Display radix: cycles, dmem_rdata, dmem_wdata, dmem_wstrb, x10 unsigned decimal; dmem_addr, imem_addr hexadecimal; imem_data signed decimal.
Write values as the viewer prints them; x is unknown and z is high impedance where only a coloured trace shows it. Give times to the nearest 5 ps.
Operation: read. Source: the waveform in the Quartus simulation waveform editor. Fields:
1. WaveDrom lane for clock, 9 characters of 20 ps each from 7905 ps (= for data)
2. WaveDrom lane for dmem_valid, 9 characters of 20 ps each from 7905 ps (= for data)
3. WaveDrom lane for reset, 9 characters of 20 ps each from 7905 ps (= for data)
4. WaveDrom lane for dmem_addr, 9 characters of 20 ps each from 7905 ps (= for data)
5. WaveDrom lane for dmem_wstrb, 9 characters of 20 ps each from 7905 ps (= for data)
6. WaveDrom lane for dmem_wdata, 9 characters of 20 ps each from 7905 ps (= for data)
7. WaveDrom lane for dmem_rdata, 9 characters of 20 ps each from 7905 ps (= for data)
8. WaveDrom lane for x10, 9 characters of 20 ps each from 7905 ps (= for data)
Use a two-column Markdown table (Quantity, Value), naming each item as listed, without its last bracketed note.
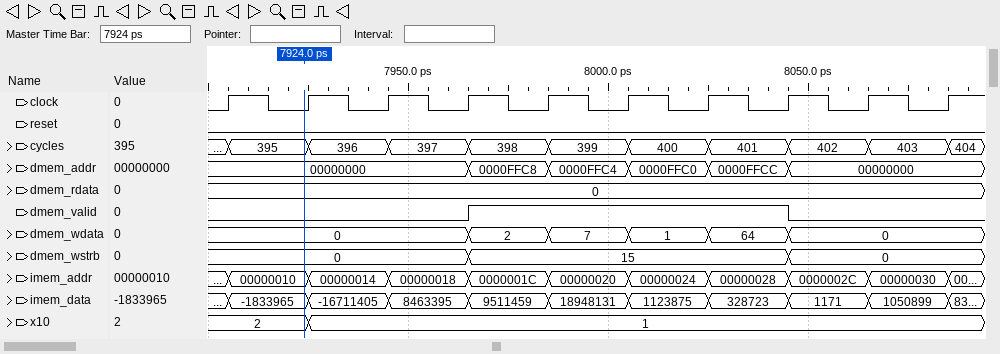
| Quantity | Value |
|---|---|
| WaveDrom lane for clock, 9 characters of 20 ps each from 7905 ps | {name: 'clock', wave: 'p........'} |
| WaveDrom lane for dmem_valid, 9 characters of 20 ps each from 7905 ps | {name: 'dmem_valid', wave: '0..1...0.'} |
| WaveDrom lane for reset, 9 characters of 20 ps each from 7905 ps | {name: 'reset', wave: '0........'} |
| WaveDrom lane for dmem_addr, 9 characters of 20 ps each from 7905 ps | {name: 'dmem_addr', wave: '=..=====.', data: '00000000 0000FFC8 0000FFC4 0000FFC0 0000FFCC 00000000'} |
| WaveDrom lane for dmem_wstrb, 9 characters of 20 ps each from 7905 ps | {name: 'dmem_wstrb', wave: '=..=...=.', data: '0 15 0'} |
| WaveDrom lane for dmem_wdata, 9 characters of 20 ps each from 7905 ps | {name: 'dmem_wdata', wave: '=..=====.', data: '0 2 7 1 64 0'} |
| WaveDrom lane for dmem_rdata, 9 characters of 20 ps each from 7905 ps | {name: 'dmem_rdata', wave: '=........', data: '0'} |
| WaveDrom lane for x10, 9 characters of 20 ps each from 7905 ps | {name: 'x10', wave: '==.......', data: '2 1'} |
